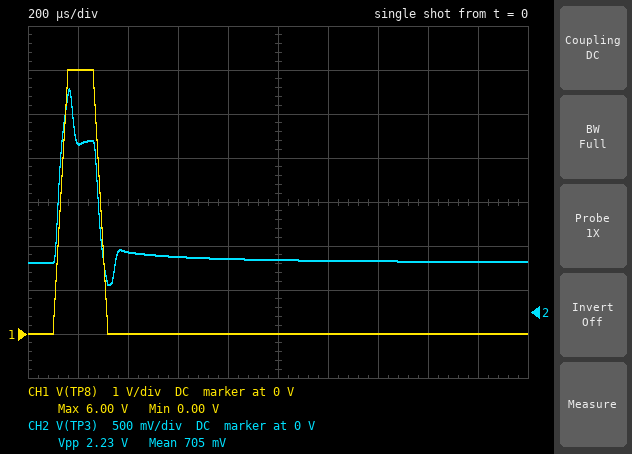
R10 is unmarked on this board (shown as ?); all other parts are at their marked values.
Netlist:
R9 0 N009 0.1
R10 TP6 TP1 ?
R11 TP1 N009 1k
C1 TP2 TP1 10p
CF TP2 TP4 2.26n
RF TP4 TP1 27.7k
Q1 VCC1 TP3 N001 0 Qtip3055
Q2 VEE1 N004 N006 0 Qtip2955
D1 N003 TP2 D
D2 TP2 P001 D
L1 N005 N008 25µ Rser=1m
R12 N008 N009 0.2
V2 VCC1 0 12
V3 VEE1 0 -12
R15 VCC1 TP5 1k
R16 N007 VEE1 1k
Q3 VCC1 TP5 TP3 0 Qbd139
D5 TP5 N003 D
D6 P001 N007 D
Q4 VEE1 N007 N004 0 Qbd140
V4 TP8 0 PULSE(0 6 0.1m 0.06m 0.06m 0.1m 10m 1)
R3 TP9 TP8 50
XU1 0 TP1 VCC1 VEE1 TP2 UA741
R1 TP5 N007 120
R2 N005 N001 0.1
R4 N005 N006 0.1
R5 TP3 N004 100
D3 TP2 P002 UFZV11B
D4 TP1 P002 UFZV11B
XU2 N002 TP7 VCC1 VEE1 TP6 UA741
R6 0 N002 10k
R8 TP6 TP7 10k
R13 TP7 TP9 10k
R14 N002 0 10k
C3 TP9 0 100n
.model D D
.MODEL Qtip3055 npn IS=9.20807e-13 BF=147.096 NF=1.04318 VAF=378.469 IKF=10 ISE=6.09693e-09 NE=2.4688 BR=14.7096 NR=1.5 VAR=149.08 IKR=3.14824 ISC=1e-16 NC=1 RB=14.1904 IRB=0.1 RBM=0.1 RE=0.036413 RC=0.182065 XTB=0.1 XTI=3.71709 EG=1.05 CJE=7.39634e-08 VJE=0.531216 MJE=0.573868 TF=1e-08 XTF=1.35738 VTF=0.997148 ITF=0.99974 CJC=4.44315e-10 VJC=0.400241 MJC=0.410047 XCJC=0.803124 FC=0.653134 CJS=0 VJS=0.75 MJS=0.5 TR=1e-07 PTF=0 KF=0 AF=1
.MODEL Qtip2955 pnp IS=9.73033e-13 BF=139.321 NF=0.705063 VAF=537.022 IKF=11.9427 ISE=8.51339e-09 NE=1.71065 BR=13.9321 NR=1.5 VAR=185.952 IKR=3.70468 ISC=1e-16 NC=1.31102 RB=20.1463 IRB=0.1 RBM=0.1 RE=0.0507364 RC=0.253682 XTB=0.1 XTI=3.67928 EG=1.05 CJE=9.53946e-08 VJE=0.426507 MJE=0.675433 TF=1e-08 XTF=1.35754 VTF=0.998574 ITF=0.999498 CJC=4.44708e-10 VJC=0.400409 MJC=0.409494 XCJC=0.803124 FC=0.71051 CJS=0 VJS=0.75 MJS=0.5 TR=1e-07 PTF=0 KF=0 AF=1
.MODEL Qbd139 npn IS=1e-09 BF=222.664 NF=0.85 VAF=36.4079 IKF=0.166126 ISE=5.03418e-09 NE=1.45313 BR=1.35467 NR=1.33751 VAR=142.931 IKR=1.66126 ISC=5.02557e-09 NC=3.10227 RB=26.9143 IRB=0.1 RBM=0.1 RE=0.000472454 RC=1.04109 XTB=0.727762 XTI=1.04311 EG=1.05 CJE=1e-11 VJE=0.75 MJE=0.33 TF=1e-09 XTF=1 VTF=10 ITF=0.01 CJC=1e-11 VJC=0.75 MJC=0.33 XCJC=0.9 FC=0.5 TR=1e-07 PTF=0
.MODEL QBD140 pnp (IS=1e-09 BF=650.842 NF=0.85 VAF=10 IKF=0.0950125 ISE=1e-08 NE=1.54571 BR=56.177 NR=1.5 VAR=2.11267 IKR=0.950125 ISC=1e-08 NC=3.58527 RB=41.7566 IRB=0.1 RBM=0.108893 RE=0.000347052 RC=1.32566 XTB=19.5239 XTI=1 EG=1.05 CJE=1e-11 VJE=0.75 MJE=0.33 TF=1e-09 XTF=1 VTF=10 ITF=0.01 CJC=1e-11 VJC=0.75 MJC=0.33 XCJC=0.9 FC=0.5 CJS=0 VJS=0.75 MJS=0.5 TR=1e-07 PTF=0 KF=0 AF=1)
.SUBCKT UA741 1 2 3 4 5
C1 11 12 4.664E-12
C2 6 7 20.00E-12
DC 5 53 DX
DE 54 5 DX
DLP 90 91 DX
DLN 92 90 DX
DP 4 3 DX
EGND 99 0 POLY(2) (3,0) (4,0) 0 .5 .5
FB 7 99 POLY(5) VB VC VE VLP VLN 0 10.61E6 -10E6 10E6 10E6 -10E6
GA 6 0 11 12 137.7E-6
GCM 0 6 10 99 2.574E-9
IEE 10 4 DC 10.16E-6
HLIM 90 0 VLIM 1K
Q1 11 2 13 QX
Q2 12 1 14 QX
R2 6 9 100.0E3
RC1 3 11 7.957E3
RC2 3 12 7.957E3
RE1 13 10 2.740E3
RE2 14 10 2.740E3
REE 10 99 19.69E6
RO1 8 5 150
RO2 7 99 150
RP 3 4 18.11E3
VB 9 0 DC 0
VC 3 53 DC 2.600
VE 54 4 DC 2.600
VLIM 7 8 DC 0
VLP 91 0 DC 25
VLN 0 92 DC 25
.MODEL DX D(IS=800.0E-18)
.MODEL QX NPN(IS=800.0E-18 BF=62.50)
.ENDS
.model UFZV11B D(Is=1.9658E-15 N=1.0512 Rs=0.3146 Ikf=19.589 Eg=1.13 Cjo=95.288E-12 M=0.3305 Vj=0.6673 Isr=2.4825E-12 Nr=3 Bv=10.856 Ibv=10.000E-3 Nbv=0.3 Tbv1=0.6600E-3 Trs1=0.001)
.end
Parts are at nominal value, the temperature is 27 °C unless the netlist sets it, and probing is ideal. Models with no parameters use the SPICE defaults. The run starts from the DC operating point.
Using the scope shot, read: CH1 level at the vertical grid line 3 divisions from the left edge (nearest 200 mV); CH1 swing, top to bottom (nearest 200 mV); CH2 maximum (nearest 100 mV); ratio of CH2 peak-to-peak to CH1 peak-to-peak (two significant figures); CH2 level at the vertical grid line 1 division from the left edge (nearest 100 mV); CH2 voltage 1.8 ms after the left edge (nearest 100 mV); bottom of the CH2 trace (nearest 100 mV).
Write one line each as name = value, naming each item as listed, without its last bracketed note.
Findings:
CH1 level at the vertical grid line 3 divisions from the left edge = 0 V
CH1 swing, top to bottom = 6.0 V
CH2 maximum = 2.5 V
ratio of CH2 peak-to-peak to CH1 peak-to-peak = 0.37
CH2 level at the vertical grid line 1 division from the left edge = 1.9 V
CH2 voltage 1.8 ms after the left edge = 600 mV
bottom of the CH2 trace = 300 mV
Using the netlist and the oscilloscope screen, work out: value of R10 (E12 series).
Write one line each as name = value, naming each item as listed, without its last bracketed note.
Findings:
value of R10 = 27 kΩ
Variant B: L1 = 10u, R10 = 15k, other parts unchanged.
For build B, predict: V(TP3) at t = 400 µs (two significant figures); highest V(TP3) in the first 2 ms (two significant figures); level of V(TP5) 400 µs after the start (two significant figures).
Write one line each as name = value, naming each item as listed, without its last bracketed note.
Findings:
V(TP3) at t = 400 µs = 760 mV
highest V(TP3) in the first 2 ms = 3.1 V
level of V(TP5) 400 µs after the start = 1.1 V
